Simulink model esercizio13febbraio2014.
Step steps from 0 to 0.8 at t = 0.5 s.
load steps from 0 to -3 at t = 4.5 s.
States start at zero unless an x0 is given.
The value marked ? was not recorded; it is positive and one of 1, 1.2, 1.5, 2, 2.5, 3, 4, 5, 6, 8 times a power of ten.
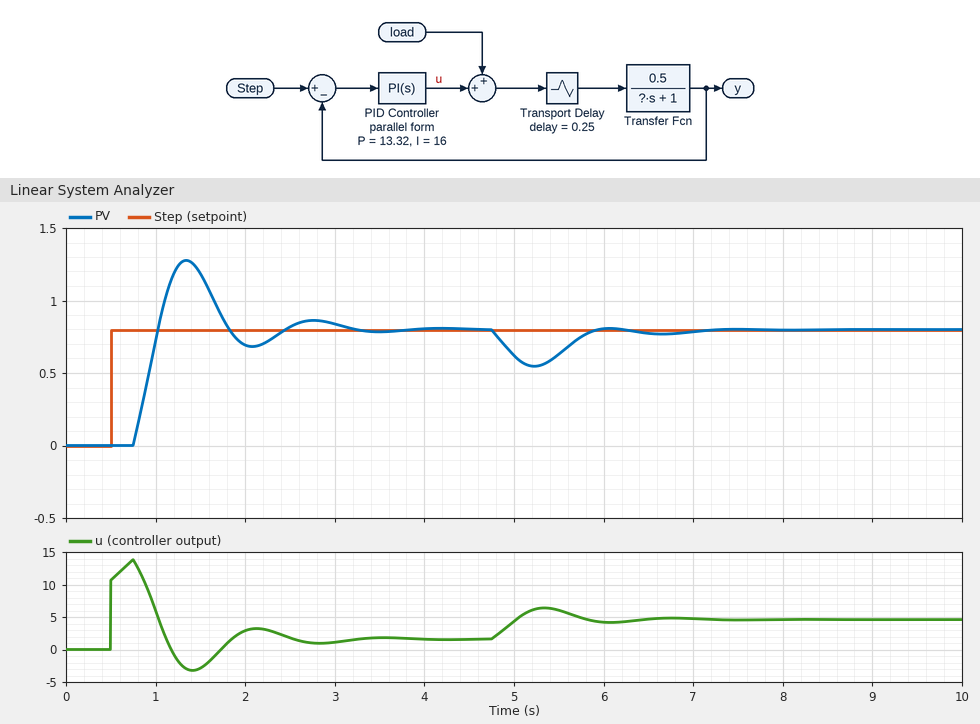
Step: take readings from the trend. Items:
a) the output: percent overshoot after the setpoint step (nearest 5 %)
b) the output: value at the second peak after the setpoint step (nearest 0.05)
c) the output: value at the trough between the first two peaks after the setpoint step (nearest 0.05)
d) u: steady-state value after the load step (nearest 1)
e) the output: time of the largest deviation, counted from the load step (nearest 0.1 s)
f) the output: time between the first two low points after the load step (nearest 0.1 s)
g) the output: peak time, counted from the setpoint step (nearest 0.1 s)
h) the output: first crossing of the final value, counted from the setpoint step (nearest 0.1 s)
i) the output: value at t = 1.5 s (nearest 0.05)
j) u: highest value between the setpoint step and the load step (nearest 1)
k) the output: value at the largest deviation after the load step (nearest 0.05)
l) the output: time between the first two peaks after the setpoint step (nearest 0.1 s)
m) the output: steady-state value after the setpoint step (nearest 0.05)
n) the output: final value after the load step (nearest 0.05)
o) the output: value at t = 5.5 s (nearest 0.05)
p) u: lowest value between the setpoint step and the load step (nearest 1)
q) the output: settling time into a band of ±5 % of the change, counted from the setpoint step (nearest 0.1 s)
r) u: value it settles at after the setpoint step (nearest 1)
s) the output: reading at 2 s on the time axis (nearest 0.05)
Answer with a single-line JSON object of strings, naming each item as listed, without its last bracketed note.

{"the output: percent overshoot after the setpoint step": "60 %", "the output: value at the second peak after the setpoint step": "0.85", "the output: value at the trough between the first two peaks after the setpoint step": "0.70", "u: steady-state value after the load step": "5", "the output: time of the largest deviation, counted from the load step": "0.7 s", "the output: time between the first two low points after the load step": "1.4 s", "the output: peak time, counted from the setpoint step": "0.8 s", "the output: first crossing of the final value, counted from the setpoint step": "0.5 s", "the output: value at t = 1.5 s": "1.20", "u: highest value between the setpoint step and the load step": "14", "the output: value at the largest deviation after the load step": "0.55", "the output: time between the first two peaks after the setpoint step": "1.4 s", "the output: steady-state value after the setpoint step": "0.80", "the output: final value after the load step": "0.80", "the output: value at t = 5.5 s": "0.65", "u: lowest value between the setpoint step and the load step": "-3", "the output: settling time into a band of ±5 % of the change, counted from the setpoint step": "2.5 s", "u: value it settles at after the setpoint step": "2", "the output: reading at 2 s on the time axis": "0.70"}
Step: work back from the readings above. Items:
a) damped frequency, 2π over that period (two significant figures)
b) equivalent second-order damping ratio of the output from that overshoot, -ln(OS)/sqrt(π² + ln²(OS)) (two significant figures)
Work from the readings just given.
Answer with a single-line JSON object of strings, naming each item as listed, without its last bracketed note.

{"damped frequency, 2π over that period": "4.5 rad/s", "equivalent second-order damping ratio of the output from that overshoot, -ln(OS)/sqrt(π² + ln²(OS))": "0.16"}
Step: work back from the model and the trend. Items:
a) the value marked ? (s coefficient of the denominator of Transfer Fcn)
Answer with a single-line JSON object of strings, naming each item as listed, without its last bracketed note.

{"the value marked ?": "2"}
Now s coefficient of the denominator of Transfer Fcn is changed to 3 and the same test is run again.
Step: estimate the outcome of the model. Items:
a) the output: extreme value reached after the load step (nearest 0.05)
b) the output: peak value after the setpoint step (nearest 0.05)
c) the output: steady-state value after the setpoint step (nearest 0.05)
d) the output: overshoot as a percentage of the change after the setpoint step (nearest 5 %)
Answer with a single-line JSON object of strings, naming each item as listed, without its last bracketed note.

{"the output: extreme value reached after the load step": "0.60", "the output: peak value after the setpoint step": "1.15", "the output: steady-state value after the setpoint step": "0.80", "the output: overshoot as a percentage of the change after the setpoint step": "40 %"}
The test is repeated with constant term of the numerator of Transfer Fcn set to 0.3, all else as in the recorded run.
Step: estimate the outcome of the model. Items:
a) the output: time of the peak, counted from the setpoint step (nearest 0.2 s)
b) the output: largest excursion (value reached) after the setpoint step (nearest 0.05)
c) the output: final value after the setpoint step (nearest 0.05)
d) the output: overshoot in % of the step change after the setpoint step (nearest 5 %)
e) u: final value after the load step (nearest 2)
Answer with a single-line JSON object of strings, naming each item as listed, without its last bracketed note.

{"the output: time of the peak, counted from the setpoint step": "1.2 s", "the output: largest excursion (value reached) after the setpoint step": "1.05", "the output: final value after the setpoint step": "0.80", "the output: overshoot in % of the step change after the setpoint step": "30 %", "u: final value after the load step": "6"}
